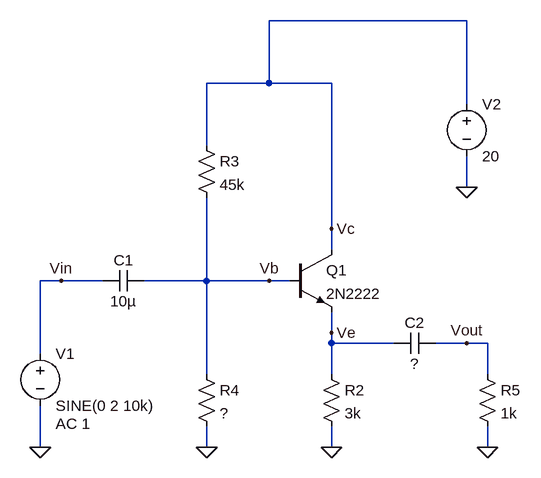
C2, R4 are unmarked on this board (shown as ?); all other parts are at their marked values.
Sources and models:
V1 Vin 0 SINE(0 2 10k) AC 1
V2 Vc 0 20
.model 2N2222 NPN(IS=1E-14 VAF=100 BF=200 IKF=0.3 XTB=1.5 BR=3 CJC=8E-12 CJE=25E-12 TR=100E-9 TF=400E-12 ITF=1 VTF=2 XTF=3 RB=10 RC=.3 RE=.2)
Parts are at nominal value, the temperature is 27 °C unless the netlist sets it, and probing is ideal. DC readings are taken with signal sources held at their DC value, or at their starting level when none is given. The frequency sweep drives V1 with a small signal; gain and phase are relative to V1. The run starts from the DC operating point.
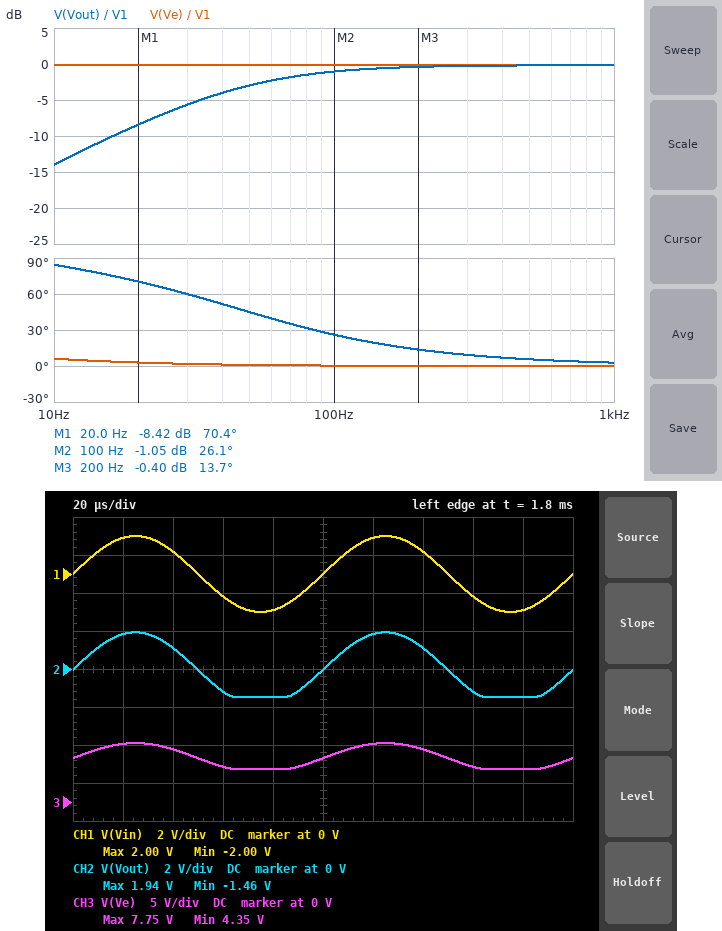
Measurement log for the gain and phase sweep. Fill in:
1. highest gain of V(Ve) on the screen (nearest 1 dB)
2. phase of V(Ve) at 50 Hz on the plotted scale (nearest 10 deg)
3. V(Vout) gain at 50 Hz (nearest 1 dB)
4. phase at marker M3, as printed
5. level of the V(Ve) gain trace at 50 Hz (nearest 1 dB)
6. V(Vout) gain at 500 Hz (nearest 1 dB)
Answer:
0 dB
0 deg
-3 dB
13.7 deg
0 dB
0 dB
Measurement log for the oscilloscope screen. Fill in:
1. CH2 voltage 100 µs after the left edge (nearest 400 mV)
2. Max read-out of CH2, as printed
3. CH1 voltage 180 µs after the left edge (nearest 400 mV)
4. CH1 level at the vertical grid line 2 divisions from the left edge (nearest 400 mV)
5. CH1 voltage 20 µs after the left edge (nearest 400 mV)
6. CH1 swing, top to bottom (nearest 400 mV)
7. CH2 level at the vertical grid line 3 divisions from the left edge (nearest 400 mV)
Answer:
0 V
1.94 V
-2.0 V
1.2 V
2.0 V
4.0 V
-1.2 V
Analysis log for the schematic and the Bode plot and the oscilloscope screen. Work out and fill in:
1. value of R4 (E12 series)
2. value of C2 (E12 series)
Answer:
22 kΩ
3.3 µF
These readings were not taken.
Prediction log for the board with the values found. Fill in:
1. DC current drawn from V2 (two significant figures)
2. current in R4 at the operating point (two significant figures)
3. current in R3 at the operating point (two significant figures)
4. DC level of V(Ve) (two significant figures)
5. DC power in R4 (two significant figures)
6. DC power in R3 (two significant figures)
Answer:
2.2 mA
290 µA
300 µA
5.8 V
1.9 mW
4.1 mW
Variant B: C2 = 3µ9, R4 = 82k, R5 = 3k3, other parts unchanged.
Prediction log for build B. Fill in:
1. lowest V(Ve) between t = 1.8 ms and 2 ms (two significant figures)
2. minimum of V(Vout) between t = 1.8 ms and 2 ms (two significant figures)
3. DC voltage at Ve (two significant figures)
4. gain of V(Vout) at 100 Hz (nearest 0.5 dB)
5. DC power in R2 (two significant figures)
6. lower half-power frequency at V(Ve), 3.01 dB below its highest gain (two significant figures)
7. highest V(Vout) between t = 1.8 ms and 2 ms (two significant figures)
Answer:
9.7 V
-2.0 V
12 V
0 dB
46 mW
570 mHz
2.0 V
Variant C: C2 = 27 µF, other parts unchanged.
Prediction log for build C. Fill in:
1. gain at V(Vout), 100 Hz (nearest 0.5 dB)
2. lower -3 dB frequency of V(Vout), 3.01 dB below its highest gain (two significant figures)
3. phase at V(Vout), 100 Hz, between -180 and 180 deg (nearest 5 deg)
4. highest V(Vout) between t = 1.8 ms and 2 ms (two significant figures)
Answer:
0 dB
6.1 Hz
5 deg
2.0 V
